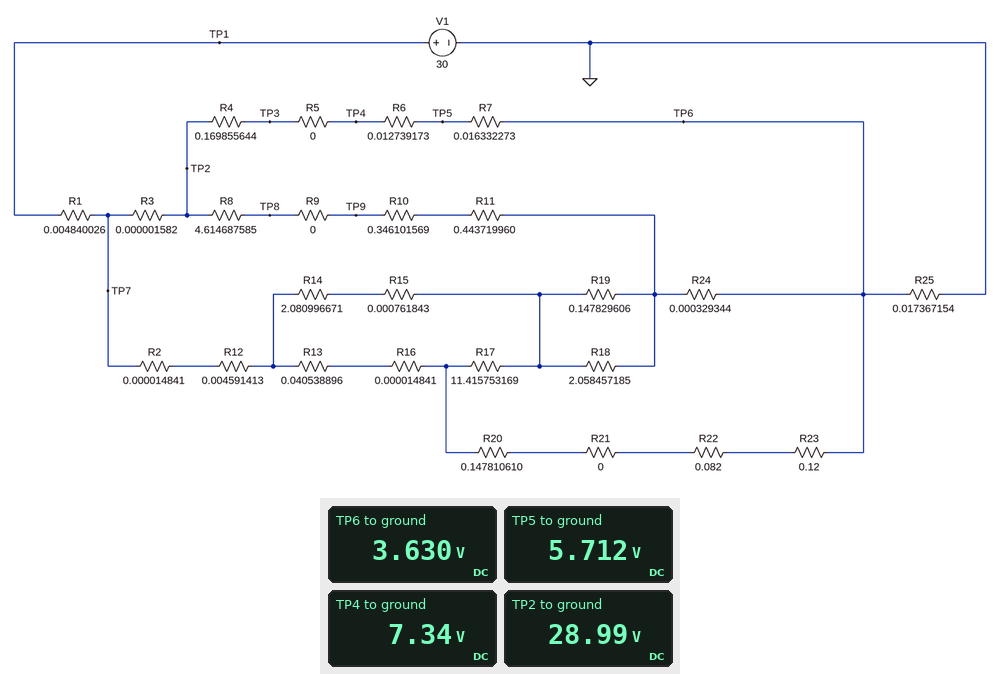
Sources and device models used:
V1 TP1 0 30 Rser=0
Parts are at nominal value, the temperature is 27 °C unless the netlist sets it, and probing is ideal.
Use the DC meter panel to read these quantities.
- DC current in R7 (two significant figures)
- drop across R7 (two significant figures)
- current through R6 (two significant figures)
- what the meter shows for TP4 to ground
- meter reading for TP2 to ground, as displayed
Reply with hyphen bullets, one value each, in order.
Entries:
- 130 A
- 2.1 V
- 130 A
- 7.34 V
- 28.99 V
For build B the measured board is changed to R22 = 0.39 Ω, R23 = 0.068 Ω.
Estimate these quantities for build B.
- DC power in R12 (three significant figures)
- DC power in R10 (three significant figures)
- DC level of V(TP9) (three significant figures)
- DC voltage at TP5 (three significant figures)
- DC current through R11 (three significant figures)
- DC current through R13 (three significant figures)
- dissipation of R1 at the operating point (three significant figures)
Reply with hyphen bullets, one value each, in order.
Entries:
- 12.8 W
- 7.91 W
- 7.04 V
- 5.38 V
- 4.78 A
- 41.4 A
- 170 W
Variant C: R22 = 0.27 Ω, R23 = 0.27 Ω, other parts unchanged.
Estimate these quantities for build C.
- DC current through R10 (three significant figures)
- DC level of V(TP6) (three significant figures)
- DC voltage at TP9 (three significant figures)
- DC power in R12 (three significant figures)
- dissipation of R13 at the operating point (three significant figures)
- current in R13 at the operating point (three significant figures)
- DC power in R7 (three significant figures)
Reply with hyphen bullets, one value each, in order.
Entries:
- 4.80 A
- 3.19 V
- 6.98 V
- 10.8 W
- 55.9 W
- 37.1 A
- 277 W
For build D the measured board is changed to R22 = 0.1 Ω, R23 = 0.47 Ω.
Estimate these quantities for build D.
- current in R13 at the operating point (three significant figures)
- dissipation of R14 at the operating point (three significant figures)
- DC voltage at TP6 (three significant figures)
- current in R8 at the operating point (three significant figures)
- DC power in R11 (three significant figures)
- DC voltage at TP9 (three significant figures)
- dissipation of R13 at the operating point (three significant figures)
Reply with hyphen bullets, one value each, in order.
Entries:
- 35.8 A
- 274 W
- 3.17 V
- 4.80 A
- 10.2 W
- 6.97 V
- 51.9 W
